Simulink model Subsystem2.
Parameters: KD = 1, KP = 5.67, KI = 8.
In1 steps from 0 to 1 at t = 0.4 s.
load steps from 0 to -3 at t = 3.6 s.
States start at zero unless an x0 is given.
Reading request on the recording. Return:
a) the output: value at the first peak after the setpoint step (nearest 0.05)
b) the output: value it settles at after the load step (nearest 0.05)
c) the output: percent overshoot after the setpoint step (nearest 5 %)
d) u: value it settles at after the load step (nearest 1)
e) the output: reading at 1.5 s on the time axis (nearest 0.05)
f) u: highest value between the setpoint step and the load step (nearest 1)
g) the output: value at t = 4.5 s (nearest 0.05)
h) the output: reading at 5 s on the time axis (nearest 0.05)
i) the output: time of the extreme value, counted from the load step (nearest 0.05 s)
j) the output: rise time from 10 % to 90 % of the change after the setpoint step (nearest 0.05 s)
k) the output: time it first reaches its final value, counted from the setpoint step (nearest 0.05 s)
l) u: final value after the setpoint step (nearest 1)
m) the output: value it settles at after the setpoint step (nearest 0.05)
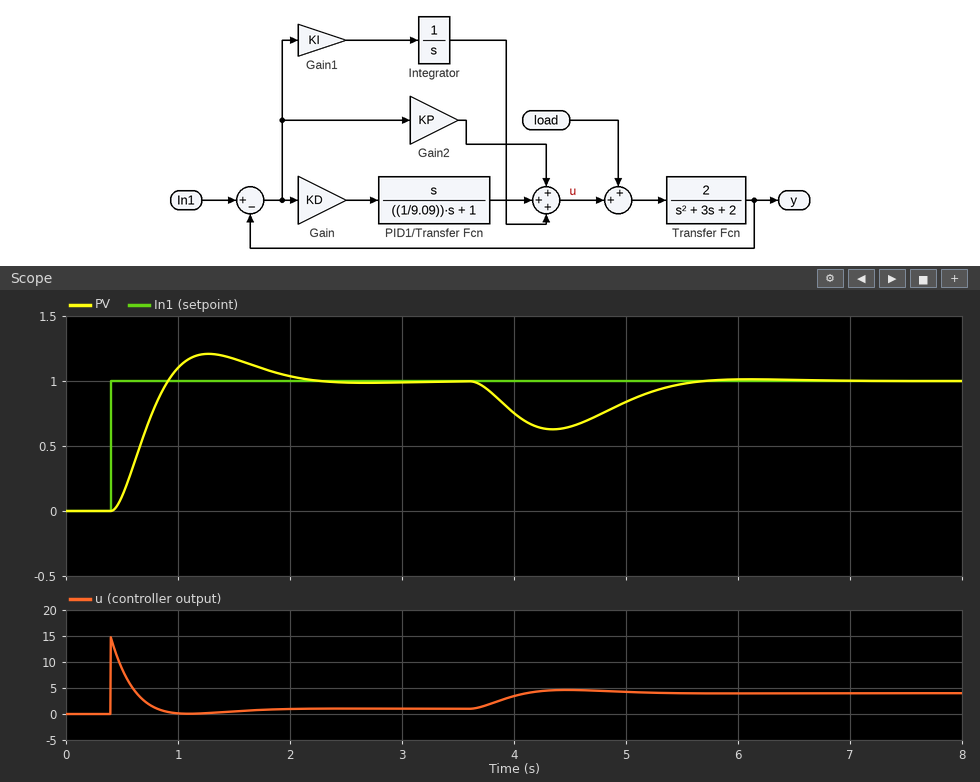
1.20
1.00
20 %
4
1.15
15
0.65
0.85
0.75 s
0.35 s
0.50 s
1
1.00
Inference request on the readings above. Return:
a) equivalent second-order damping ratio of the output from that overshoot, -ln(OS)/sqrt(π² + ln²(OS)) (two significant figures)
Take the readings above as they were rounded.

0.46
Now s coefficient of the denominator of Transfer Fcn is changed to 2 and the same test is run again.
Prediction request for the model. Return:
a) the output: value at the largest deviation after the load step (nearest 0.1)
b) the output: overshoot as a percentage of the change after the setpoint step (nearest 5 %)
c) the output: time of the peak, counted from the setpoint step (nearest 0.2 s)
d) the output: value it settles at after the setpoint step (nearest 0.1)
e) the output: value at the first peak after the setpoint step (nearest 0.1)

0.6
30 %
0.8 s
1.0
1.3
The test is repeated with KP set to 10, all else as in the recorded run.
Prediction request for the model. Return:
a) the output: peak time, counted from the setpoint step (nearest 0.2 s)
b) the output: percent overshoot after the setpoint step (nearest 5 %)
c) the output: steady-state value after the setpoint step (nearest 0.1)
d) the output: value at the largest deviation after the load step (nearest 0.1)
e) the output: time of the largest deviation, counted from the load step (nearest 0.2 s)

0.6 s
25 %
1.0
0.7
0.6 s
